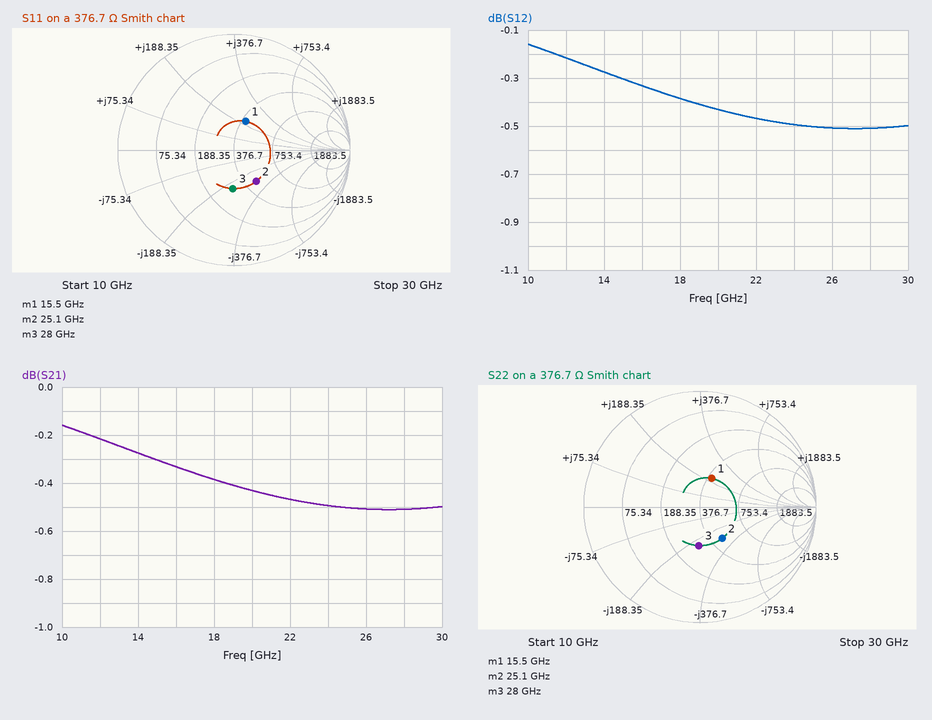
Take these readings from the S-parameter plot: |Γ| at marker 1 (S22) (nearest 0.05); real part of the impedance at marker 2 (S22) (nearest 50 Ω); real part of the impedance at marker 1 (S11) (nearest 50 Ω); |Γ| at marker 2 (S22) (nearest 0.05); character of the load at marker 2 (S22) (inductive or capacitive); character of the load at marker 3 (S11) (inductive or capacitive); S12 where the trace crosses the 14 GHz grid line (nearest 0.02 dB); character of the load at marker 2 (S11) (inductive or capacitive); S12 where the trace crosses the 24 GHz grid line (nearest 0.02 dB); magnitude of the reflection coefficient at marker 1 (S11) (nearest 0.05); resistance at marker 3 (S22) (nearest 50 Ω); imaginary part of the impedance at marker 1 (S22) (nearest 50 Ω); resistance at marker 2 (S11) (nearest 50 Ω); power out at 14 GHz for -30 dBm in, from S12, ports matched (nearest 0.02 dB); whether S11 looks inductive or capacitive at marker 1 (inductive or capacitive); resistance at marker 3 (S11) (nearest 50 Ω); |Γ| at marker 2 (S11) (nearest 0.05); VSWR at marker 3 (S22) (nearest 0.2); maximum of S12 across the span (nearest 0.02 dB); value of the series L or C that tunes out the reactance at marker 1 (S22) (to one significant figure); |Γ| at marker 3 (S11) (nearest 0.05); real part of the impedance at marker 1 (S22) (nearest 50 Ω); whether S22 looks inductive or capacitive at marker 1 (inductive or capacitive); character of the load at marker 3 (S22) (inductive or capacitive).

0.25
450 Ω
400 Ω
0.35
capacitive
capacitive
-0.28 dB
capacitive
-0.50 dB
0.25
300 Ω
+200 Ω
450 Ω
-30.28 dBm
inductive
300 Ω
0.35
2.0
-0.16 dB
50 fF
0.35
400 Ω
inductive
capacitive
